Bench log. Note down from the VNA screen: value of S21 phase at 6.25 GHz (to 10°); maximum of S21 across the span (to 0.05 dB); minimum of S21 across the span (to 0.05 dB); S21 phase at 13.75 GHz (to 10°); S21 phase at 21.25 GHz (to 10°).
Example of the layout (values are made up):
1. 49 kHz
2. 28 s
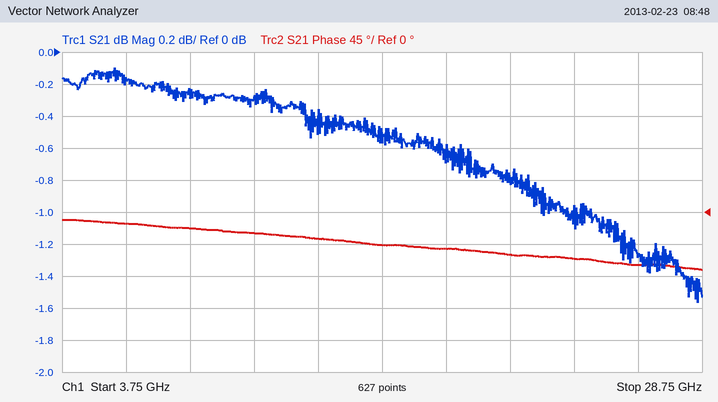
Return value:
1. -20°
2. -0.10 dB
3. -1.55 dB
4. -40°
5. -60°
